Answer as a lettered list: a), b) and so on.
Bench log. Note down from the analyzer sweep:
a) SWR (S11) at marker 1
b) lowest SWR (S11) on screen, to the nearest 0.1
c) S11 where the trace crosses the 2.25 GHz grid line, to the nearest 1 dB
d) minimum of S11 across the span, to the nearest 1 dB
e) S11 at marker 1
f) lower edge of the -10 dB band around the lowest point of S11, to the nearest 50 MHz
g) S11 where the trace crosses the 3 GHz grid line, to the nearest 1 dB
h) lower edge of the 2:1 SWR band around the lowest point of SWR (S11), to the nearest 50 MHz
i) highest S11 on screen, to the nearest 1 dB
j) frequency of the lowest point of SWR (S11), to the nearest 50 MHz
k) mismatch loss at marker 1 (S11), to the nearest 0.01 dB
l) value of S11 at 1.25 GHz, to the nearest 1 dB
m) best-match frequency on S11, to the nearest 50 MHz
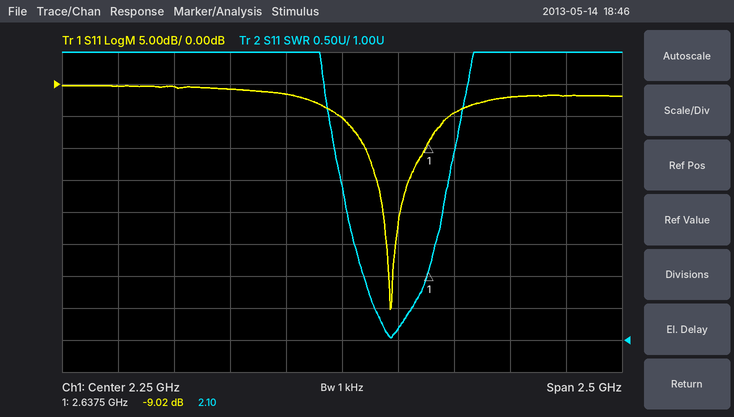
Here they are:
a) 2.10
b) 1.0
c) -5 dB
d) -35 dB
e) -9.02 dB
f) 2.35 GHz
g) -2 dB
h) 2.35 GHz
i) 0 dB
j) 2.45 GHz
k) 0.58 dB
l) 0 dB
m) 2.45 GHz
